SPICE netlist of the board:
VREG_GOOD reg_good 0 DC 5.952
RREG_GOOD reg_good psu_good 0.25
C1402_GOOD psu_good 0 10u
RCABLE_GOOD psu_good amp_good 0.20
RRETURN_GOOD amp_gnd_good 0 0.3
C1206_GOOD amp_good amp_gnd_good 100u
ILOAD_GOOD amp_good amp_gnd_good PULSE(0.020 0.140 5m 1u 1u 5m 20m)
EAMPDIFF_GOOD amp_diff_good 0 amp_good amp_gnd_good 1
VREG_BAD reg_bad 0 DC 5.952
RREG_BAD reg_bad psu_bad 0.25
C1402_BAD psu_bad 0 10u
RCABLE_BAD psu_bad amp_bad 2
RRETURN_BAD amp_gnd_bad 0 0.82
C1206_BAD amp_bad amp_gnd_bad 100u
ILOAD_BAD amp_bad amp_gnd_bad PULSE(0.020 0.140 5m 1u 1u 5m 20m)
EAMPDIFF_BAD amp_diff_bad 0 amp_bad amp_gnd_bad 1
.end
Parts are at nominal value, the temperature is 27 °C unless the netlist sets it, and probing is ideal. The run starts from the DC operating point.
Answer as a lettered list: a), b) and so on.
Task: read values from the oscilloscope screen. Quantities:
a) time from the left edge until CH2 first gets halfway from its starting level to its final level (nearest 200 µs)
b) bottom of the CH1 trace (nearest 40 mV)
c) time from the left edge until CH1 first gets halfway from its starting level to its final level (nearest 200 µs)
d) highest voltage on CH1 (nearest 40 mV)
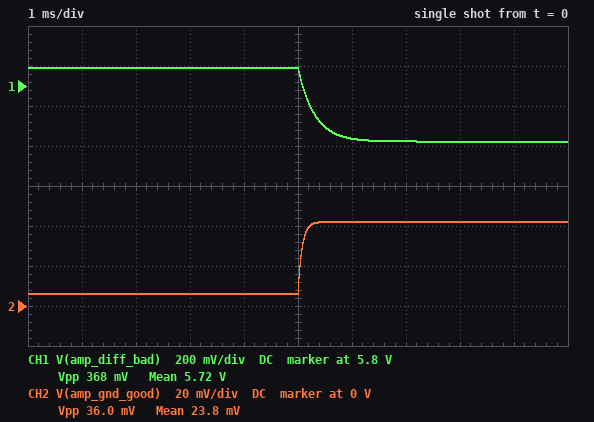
a) 5.0 ms
b) 5.52 V
c) 5.2 ms
d) 5.88 V
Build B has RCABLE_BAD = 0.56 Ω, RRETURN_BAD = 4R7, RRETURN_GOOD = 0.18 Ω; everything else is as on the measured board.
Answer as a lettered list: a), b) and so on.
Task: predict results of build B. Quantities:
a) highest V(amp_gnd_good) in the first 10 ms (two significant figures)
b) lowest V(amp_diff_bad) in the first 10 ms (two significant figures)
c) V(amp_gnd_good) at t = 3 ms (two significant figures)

a) 25 mV
b) 5.2 V
c) 3.6 mV
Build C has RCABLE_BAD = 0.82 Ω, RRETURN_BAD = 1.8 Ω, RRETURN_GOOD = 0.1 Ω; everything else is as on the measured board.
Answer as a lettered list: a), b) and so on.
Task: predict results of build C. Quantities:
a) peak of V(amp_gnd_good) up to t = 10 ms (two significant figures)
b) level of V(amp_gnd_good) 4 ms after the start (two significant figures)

a) 14 mV
b) 2.0 mV
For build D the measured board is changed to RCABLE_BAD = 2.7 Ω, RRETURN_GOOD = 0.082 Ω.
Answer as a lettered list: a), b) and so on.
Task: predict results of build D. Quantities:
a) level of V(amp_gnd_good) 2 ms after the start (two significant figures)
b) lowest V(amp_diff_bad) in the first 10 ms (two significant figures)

a) 1.6 mV
b) 5.4 V
